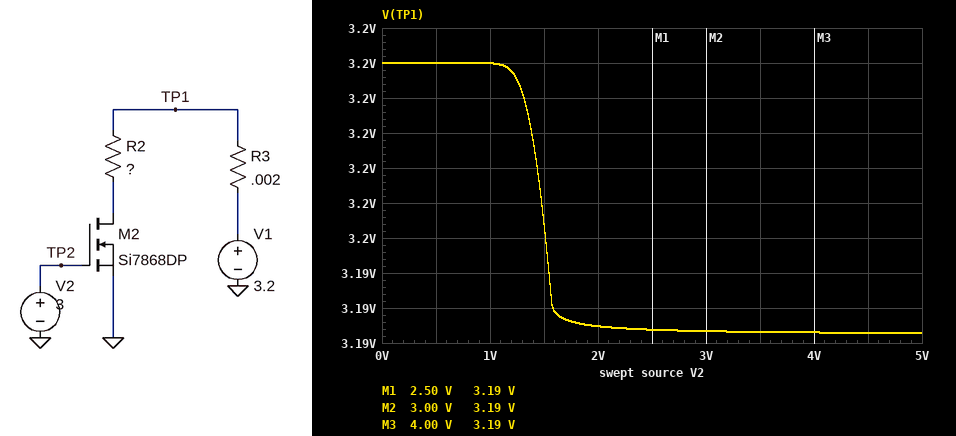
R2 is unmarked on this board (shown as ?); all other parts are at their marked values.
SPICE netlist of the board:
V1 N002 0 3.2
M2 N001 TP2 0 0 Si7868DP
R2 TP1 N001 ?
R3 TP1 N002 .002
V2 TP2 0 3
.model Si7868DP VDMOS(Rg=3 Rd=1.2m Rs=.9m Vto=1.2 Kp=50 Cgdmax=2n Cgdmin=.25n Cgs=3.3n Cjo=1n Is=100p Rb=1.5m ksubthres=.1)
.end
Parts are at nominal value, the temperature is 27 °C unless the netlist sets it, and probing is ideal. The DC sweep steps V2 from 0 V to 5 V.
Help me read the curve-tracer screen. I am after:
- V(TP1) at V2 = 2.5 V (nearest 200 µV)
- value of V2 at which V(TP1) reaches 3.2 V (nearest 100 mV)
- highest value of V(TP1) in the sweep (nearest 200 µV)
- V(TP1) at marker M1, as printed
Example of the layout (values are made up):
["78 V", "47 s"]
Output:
["3.1924 V", "1.5 V", "3.2000 V", "3.19 V"]
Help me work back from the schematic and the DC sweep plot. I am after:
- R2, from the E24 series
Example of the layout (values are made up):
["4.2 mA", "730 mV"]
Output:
["0.82 Ω"]
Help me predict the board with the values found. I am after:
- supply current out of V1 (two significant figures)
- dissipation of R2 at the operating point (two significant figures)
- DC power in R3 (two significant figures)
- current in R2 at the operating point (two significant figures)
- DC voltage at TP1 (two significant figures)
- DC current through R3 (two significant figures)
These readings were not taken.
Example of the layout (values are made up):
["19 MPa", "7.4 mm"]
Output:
["3.8 A", "12 W", "29 mW", "3.8 A", "3.2 V", "3.8 A"]
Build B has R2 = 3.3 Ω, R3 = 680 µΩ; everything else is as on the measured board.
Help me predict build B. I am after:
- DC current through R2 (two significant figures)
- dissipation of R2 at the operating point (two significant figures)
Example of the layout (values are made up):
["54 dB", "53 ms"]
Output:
["970 mA", "3.1 W"]
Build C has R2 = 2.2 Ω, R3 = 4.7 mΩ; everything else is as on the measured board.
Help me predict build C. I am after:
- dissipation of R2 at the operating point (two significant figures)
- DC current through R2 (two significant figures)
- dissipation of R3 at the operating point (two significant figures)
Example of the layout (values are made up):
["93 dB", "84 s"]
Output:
["4.6 W", "1.4 A", "9.8 mW"]
